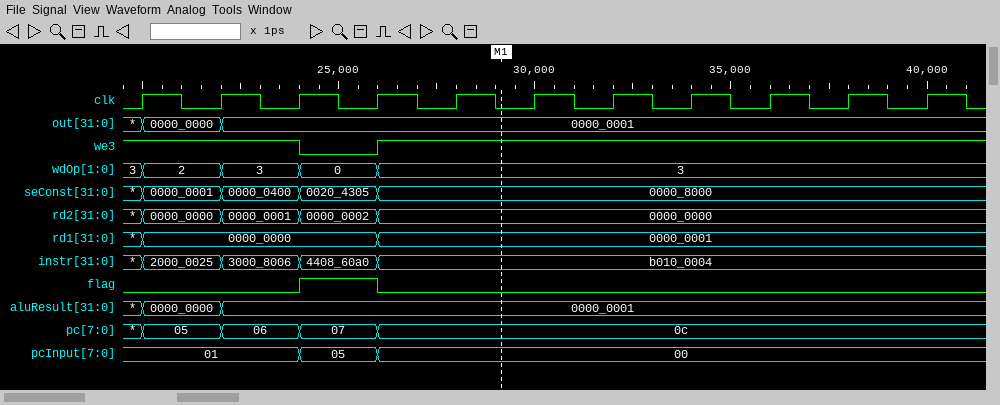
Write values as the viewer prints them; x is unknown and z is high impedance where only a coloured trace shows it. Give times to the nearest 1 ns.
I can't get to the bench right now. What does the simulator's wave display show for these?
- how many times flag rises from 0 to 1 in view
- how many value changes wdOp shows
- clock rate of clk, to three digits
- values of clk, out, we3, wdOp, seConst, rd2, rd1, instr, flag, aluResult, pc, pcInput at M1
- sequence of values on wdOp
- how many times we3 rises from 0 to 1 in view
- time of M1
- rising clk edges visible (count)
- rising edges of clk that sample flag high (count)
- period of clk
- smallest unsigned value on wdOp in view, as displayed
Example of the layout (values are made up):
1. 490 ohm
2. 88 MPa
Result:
1. 1
2. 4
3. 500 MHz
4. clk=0, out=0000_0001, we3=1, wdOp=3, seConst=0000_8000, rd2=0000_0000, rd1=0000_0001, instr=b010_0004, flag=0, aluResult=0000_0001, pc=0c, pcInput=00
5. 3, 2, 3, 0, 3
6. 1
7. 29 ns
8. 11
9. 1
10. 2 ns
11. 0
